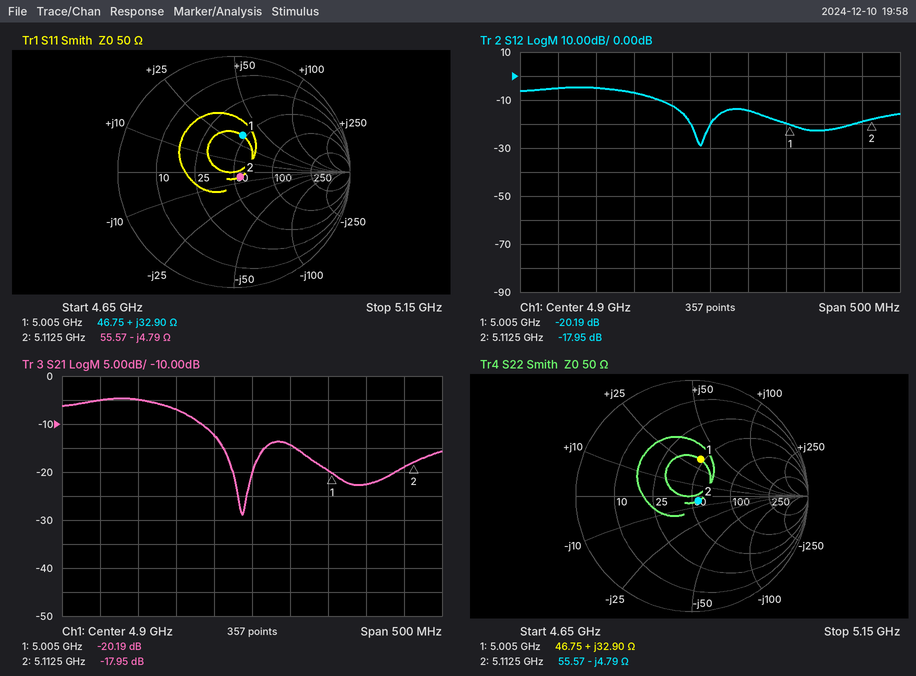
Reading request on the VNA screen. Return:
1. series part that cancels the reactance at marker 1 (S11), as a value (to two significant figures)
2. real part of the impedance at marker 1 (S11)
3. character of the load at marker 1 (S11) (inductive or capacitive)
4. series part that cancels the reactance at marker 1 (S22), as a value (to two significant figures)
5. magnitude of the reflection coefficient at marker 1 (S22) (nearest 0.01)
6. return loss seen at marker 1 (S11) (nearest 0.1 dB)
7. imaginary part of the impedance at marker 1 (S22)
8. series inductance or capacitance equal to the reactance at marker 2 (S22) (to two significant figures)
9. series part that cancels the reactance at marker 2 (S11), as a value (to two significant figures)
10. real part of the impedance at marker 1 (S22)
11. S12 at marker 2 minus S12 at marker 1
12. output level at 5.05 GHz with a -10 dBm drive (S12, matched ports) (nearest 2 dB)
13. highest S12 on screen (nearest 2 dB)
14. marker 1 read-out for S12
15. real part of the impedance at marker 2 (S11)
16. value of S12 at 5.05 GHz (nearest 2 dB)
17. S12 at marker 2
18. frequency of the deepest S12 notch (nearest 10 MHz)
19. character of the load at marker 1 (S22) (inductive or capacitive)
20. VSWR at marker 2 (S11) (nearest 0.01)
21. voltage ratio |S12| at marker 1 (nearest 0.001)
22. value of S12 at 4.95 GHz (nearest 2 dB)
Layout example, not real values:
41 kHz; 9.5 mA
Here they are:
970 fF; 46.75 Ω; inductive; 970 fF; 0.32; 9.8 dB; +32.90 Ω; 6.5 pF; 150 pH; 46.75 Ω; 2.24 dB; -32 dBm; -4 dB; -20.19 dB; 55.57 Ω; -22 dB; -17.95 dB; 4.89 GHz; inductive; 1.15; 0.098; -14 dB
